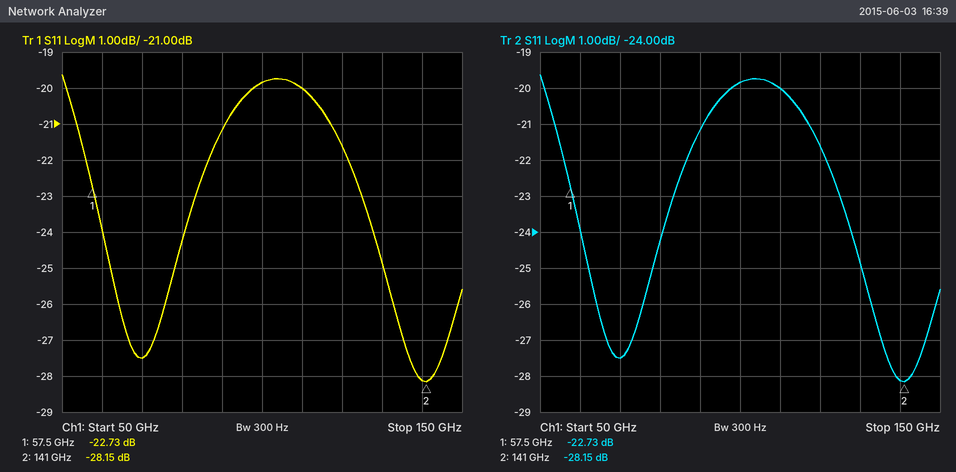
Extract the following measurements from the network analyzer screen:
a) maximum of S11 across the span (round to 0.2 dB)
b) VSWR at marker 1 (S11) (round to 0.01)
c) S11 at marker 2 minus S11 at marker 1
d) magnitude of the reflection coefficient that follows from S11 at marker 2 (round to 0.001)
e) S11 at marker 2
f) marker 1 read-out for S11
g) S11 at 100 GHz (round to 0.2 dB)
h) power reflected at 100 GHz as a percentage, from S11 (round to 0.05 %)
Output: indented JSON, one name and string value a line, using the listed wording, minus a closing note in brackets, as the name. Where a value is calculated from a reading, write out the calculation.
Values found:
{
  "maximum of S11 across the span": "-19.6 dB",
  "VSWR at marker 1 (S11)": "(1 + 0.0730)/(1 − 0.0730) ≈ 1.16",
  "S11 at marker 2 minus S11 at marker 1": "-28.15 − (-22.73) = -5.42 dB",
  "magnitude of the reflection coefficient that follows from S11 at marker 2": "10^(-28.15/20) ≈ 0.039",
  "S11 at marker 2": "-28.15 dB",
  "marker 1 read-out for S11": "-22.73 dB",
  "S11 at 100 GHz": "-19.8 dB",
  "power reflected at 100 GHz as a percentage, from S11": "10^(-19.8/10) ≈ 1.05 %"
}
